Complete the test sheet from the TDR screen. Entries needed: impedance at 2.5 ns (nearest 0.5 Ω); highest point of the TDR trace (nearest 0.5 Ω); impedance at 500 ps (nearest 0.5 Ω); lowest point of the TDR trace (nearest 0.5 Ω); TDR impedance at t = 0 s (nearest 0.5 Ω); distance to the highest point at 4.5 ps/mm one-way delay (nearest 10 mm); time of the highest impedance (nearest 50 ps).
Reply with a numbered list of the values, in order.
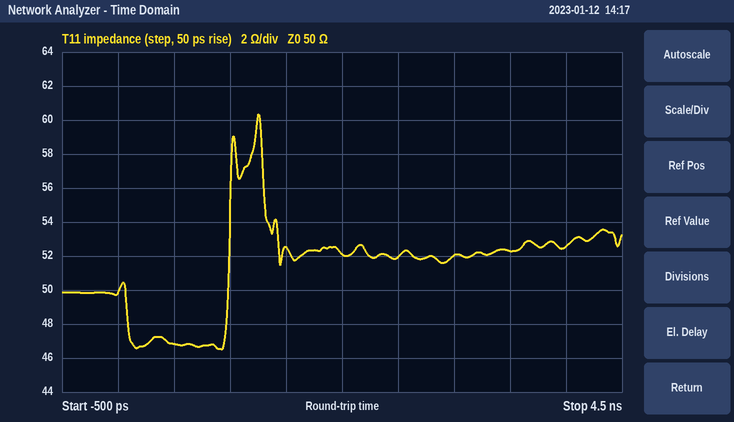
1. 52.0 Ω
2. 60.5 Ω
3. 47.0 Ω
4. 46.5 Ω
5. 50.0 Ω
6. 140 mm
7. 1.25 ns
